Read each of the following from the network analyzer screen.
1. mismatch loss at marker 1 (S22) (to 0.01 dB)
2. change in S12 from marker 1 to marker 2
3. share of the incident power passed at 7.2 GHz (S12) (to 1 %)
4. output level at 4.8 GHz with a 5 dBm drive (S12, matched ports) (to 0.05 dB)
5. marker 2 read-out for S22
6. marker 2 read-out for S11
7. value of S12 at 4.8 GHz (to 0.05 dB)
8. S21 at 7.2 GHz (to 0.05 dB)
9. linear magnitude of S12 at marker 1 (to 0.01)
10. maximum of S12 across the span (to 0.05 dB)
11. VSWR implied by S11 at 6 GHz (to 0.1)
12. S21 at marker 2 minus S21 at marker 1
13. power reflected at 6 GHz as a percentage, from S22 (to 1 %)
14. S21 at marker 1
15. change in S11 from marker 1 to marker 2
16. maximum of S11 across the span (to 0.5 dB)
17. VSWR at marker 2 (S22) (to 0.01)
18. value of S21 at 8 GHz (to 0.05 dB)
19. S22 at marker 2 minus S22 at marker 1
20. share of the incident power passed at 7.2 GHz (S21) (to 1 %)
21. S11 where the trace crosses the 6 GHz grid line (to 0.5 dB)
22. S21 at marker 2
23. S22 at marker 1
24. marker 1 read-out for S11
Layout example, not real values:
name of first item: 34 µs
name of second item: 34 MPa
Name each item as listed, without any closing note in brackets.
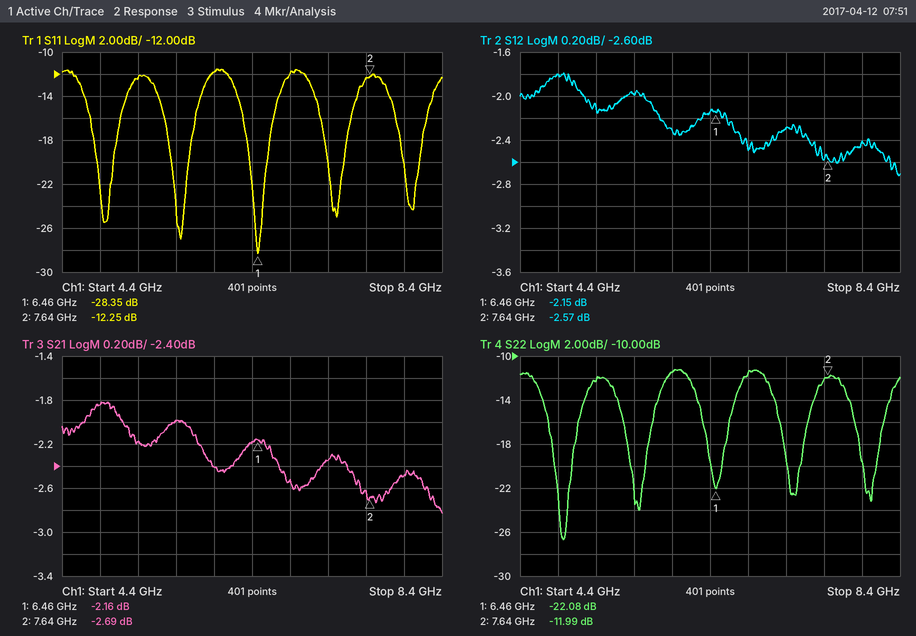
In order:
mismatch loss at marker 1 (S22): 0.03 dB
change in S12 from marker 1 to marker 2: -0.42 dB
share of the incident power passed at 7.2 GHz (S12): 59 %
output level at 4.8 GHz with a 5 dBm drive (S12, matched ports): 3.20 dBm
marker 2 read-out for S22: -11.99 dB
marker 2 read-out for S11: -12.25 dB
value of S12 at 4.8 GHz: -1.80 dB
S21 at 7.2 GHz: -2.35 dB
linear magnitude of S12 at marker 1: 0.78
maximum of S12 across the span: -1.80 dB
VSWR implied by S11 at 6 GHz: 1.7
S21 at marker 2 minus S21 at marker 1: -0.53 dB
power reflected at 6 GHz as a percentage, from S22: 7 %
S21 at marker 1: -2.16 dB
change in S11 from marker 1 to marker 2: 16.10 dB
maximum of S11 across the span: -11.5 dB
VSWR at marker 2 (S22): 1.67
value of S21 at 8 GHz: -2.50 dB
S22 at marker 2 minus S22 at marker 1: 10.09 dB
share of the incident power passed at 7.2 GHz (S21): 58 %
S11 where the trace crosses the 6 GHz grid line: -12.0 dB
S21 at marker 2: -2.69 dB
S22 at marker 1: -22.08 dB
marker 1 read-out for S11: -28.35 dB
